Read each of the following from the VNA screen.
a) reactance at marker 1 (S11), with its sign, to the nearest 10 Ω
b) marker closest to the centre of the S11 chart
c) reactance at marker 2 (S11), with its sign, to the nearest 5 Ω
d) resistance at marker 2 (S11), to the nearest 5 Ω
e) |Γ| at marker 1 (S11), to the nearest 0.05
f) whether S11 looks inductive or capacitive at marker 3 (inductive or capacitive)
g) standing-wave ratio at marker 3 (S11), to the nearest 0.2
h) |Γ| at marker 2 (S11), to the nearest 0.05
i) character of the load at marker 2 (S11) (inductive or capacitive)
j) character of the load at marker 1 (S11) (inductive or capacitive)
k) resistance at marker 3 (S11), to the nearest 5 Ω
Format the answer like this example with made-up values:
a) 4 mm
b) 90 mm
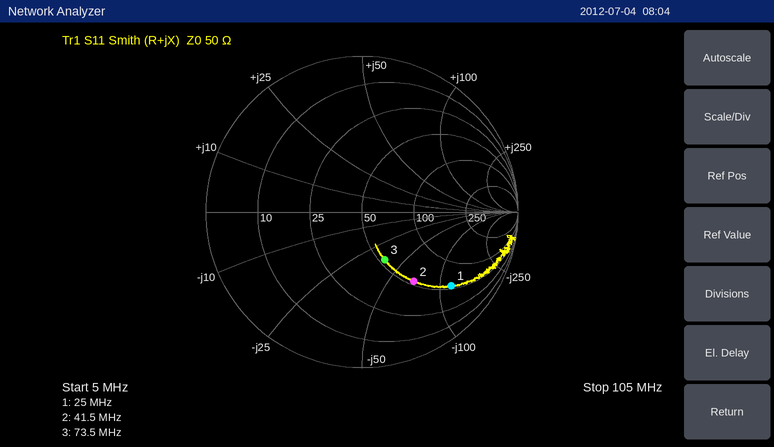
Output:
a) -120 Ω
b) marker 3
c) -70 Ω
d) 55 Ω
e) 0.75
f) capacitive
g) 2.0
h) 0.55
i) capacitive
j) capacitive
k) 55 Ω
